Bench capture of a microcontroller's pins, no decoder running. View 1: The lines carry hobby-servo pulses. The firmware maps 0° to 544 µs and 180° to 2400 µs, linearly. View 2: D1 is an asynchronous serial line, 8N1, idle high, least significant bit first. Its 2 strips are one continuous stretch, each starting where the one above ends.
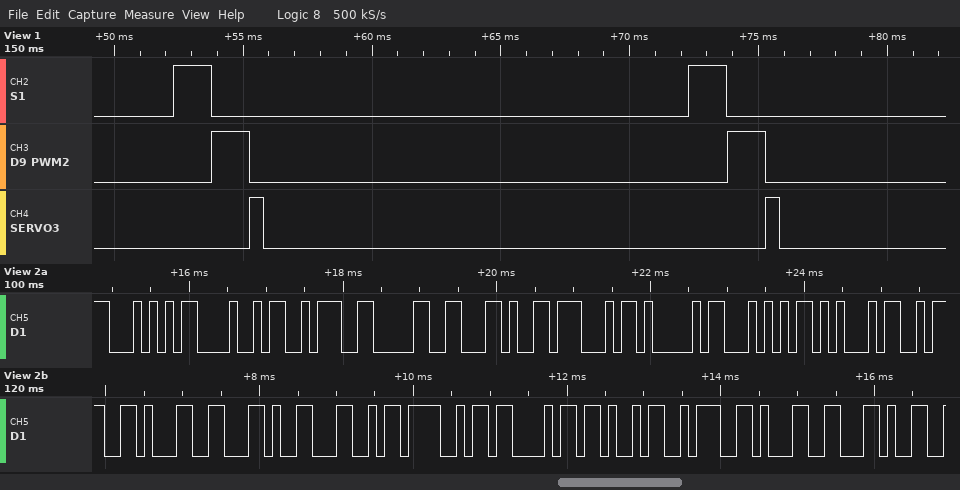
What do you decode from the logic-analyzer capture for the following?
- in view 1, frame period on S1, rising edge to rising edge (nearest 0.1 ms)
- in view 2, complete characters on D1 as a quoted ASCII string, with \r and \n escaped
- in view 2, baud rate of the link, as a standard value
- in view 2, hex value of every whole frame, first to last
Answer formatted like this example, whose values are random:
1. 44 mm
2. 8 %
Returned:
1. 20.0 ms
2. "TH:0,GATE:1,LOCK:1,"
3. 9600 baud
4. 0x54 0x48 0x3A 0x30 0x2C 0x47 0x41 0x54 0x45 0x3A 0x31 0x2C 0x4C 0x4F 0x43 0x4B 0x3A 0x31 0x2C
